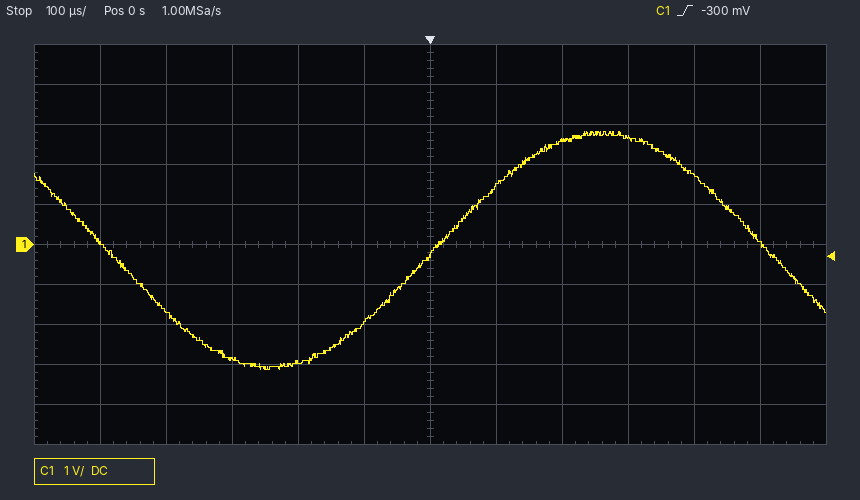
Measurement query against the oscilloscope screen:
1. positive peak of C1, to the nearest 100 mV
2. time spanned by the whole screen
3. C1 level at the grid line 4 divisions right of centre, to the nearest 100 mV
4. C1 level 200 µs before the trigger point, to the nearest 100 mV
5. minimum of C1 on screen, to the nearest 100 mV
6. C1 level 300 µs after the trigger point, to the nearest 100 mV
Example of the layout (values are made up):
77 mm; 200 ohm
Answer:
2.8 V; 1.2 ms; 1.7 V; -2.9 V; -3.1 V; 2.7 V
